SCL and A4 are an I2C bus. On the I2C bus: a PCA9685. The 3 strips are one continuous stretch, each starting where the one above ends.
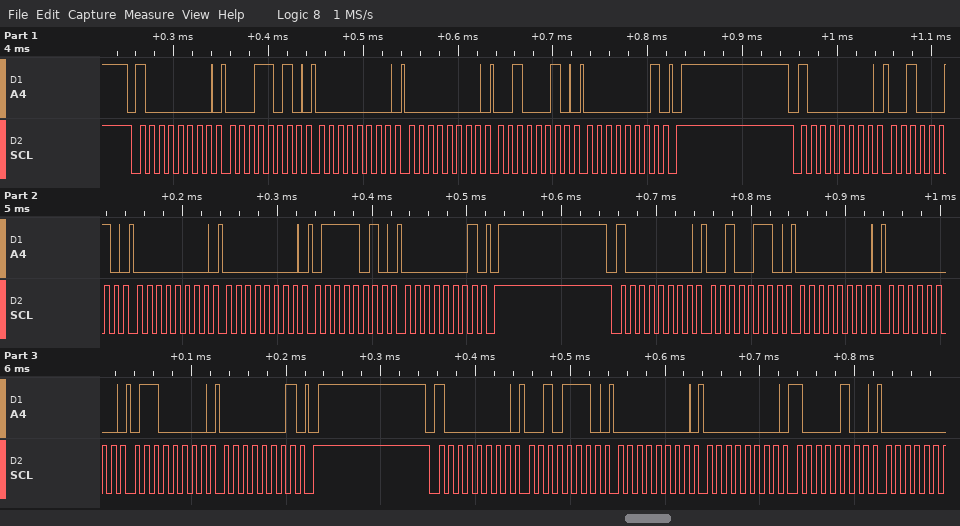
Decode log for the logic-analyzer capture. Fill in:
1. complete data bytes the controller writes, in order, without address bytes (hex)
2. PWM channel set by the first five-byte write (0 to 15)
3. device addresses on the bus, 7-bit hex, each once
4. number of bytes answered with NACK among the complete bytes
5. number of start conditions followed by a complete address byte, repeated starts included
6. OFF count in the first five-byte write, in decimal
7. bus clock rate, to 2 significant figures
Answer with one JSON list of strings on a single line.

["1A 00 00 22 01 22 00 00 7A 01 26 00 00 60 01 2E 00 00 84", "5", "0x40", "0", "4", "290", "100 kHz"]
